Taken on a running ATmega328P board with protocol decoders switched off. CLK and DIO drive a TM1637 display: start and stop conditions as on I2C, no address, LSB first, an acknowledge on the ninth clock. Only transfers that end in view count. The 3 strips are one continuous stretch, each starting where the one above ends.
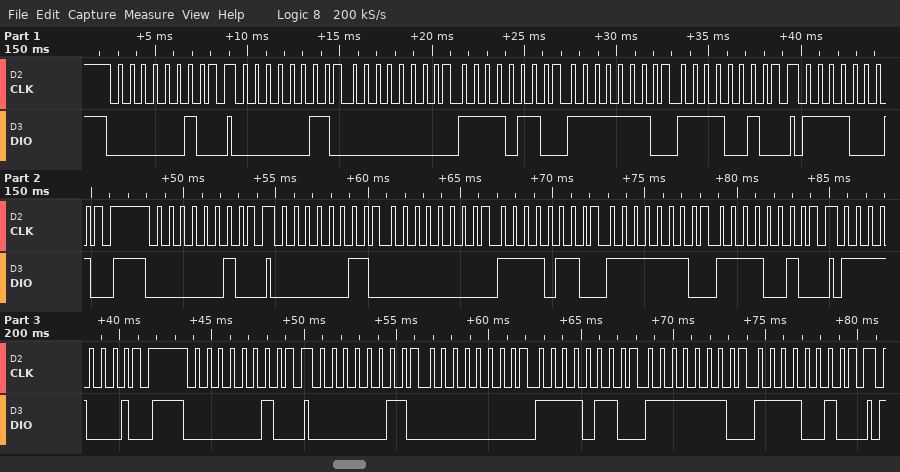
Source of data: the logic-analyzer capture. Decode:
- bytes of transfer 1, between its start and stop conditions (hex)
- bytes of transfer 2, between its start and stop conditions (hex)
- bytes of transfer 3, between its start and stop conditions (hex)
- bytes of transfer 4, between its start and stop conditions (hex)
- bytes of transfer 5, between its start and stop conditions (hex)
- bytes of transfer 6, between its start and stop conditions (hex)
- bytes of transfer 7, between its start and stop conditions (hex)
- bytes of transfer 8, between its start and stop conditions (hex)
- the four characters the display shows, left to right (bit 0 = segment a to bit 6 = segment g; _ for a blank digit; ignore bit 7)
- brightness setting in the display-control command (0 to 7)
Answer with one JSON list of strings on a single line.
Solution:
["40", "C0 00 6F 7F 4F", "8F", "40", "C0 00 6F 7F 4F", "8F", "40", "C0 00 6F 7F 4F", "_983", "7"]
